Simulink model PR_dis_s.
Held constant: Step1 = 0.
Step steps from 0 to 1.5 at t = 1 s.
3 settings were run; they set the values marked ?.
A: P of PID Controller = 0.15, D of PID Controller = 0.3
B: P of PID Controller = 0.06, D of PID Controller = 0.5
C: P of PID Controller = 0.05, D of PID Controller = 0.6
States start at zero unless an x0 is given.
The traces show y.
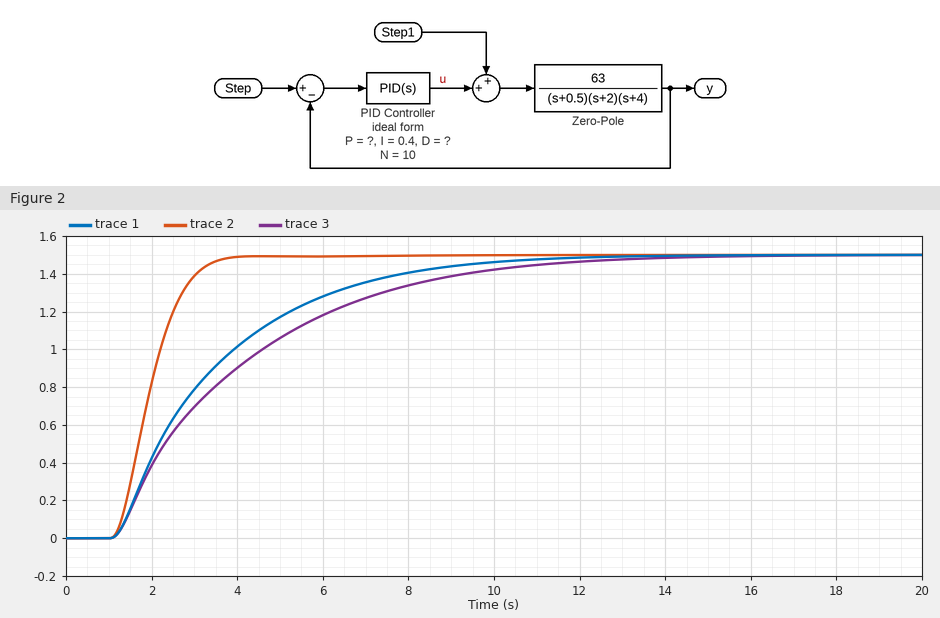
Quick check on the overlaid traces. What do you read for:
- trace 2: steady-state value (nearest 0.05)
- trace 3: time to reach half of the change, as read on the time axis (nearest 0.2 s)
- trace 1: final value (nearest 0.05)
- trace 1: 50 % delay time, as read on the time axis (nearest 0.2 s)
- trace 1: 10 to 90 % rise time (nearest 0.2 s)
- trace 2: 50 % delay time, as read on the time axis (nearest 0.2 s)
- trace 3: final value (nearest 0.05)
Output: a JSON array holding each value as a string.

["1.50", "3.2 s", "1.50", "2.8 s", "5.4 s", "2.0 s", "1.50"]
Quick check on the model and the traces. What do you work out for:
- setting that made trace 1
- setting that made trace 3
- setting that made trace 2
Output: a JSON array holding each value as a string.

["B", "C", "A"]
